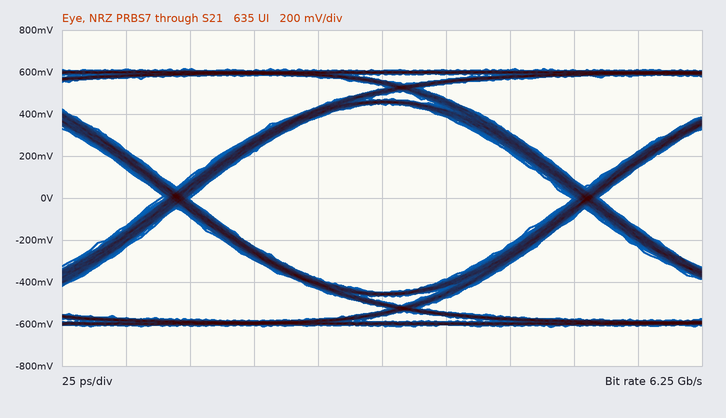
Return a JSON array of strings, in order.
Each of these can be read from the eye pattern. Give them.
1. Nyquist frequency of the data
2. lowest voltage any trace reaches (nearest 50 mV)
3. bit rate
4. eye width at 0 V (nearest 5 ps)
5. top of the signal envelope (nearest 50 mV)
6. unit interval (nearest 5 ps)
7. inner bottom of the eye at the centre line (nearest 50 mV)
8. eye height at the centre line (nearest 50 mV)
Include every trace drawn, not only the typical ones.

["3.125 GHz", "-600 mV", "6.25 Gb/s", "150 ps", "600 mV", "160 ps", "-450 mV", "900 mV"]
